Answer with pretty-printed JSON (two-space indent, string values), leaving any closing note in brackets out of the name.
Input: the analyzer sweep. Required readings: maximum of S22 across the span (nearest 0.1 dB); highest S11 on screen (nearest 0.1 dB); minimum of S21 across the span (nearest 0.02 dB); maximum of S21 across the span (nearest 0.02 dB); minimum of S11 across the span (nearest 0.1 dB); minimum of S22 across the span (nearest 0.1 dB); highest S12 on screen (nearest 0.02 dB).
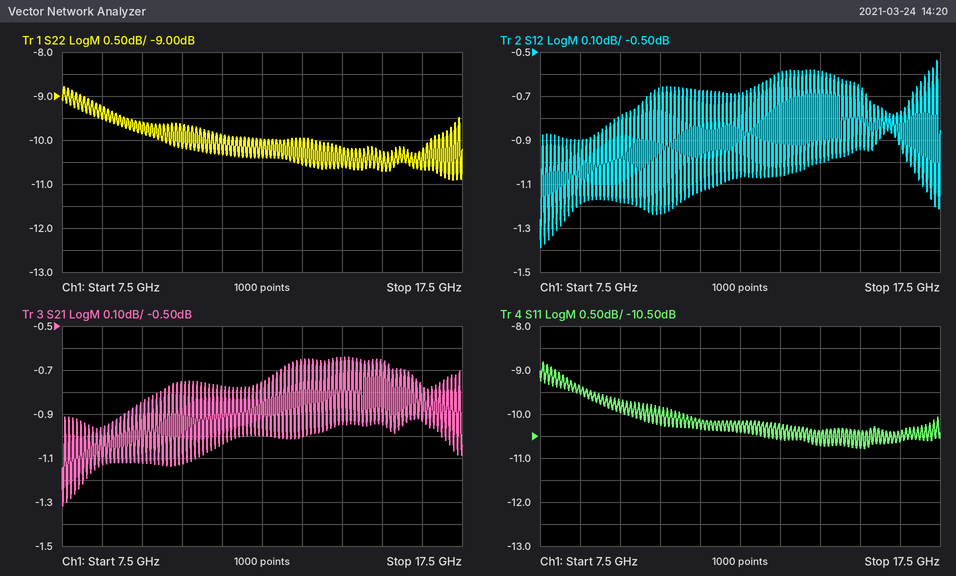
{
  "maximum of S22 across the span": "-8.8 dB",
  "highest S11 on screen": "-8.8 dB",
  "minimum of S21 across the span": "-1.32 dB",
  "maximum of S21 across the span": "-0.64 dB",
  "minimum of S11 across the span": "-10.8 dB",
  "minimum of S22 across the span": "-10.9 dB",
  "highest S12 on screen": "-0.54 dB"
}
